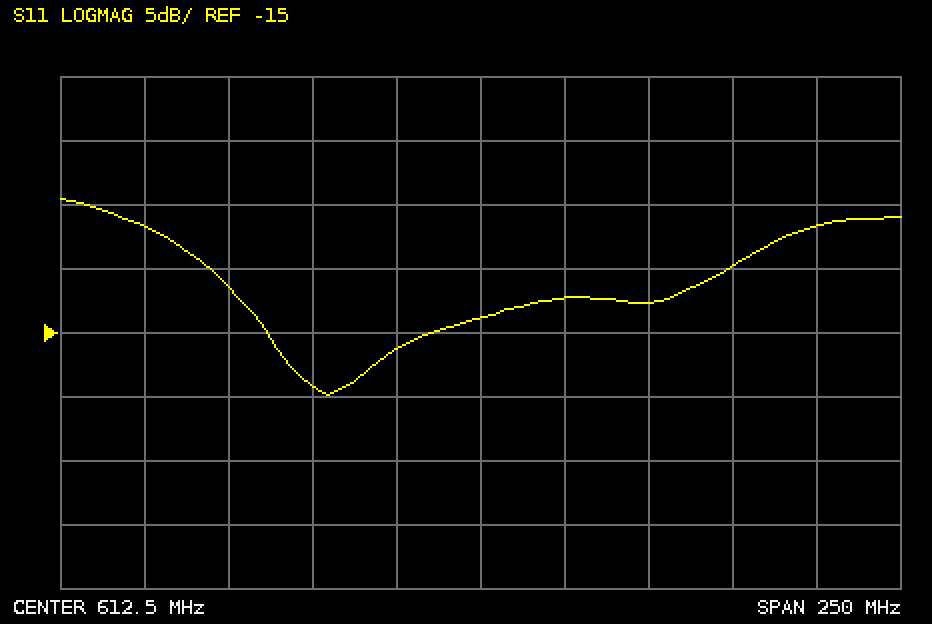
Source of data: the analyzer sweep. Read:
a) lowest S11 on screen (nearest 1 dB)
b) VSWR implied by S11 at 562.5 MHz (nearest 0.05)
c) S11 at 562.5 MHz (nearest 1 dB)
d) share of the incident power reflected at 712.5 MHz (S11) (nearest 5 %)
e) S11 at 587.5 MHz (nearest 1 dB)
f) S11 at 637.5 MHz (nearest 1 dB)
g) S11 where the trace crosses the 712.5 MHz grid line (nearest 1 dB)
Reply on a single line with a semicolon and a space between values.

-20 dB; 1.25; -19 dB; 20 %; -16 dB; -12 dB; -7 dB
